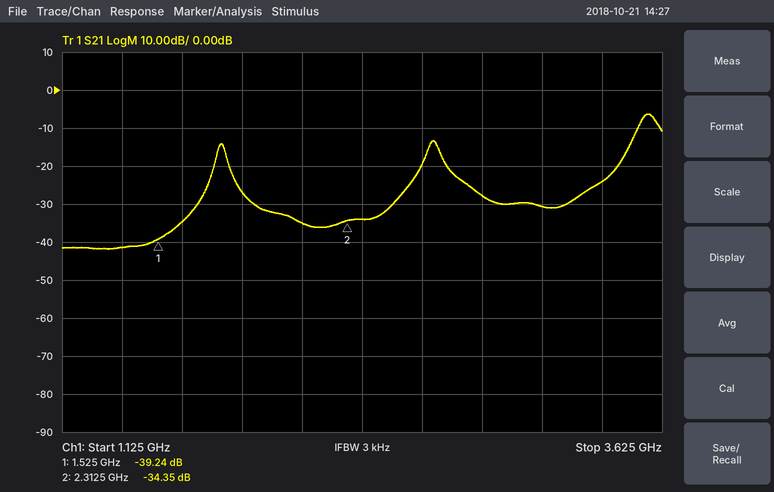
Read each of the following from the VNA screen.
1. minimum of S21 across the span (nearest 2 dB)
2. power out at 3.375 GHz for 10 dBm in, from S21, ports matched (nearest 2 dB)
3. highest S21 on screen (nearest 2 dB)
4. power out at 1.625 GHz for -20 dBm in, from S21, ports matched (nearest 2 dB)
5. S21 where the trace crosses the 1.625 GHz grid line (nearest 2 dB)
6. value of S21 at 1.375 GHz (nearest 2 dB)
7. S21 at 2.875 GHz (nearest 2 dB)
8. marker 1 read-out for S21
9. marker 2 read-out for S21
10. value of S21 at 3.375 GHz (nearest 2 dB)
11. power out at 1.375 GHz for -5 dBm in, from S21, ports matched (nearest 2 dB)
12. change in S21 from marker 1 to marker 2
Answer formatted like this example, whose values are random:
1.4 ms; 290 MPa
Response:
-42 dB; -14 dBm; -6 dB; -54 dBm; -34 dB; -42 dB; -28 dB; -39.24 dB; -34.35 dB; -24 dB; -46 dBm; 4.89 dB
